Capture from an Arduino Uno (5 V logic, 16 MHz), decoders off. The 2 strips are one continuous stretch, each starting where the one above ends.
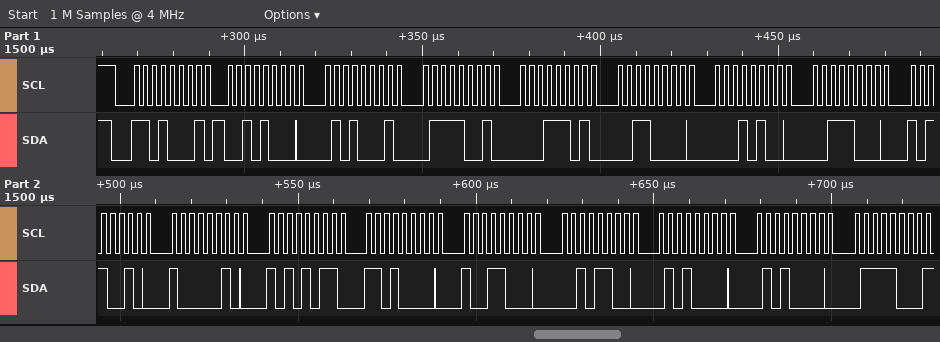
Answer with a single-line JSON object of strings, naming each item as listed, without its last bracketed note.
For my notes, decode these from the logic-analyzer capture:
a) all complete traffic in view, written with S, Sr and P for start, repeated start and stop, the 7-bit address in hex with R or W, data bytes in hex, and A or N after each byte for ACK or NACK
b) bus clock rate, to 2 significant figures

{"all complete traffic in view, written with S, Sr and P for start, repeated start and stop, the 7-bit address in hex with R or W, data bytes in hex, and A or N after each byte for ACK or NACK": "S 68R A 28 A 51 A 79 A 1D A 30 A 14 A 38 A B2 A 82 A AB A D0 A 98 A 2C A 50 A 50 A 78 N", "bus clock rate, to 2 significant figures": "400 kHz"}
